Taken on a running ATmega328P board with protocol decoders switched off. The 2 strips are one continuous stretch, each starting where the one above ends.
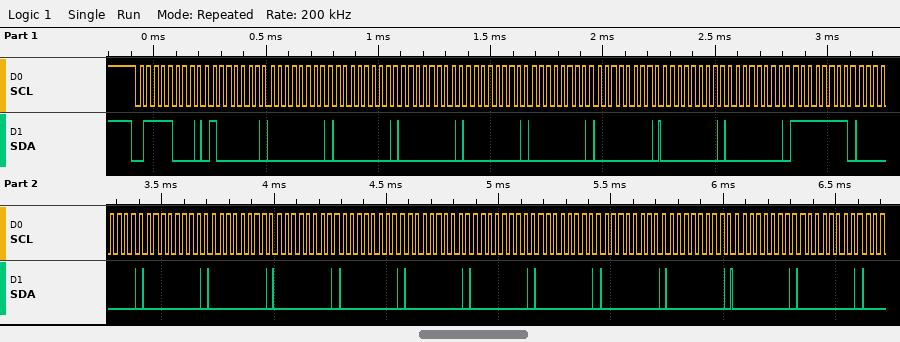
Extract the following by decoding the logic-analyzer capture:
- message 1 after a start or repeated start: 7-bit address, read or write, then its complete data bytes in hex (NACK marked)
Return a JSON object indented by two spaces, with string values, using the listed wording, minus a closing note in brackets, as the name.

{
  "message 1 after a start or repeated start: 7-bit address, read or write, then its complete data bytes in hex": "0x3C write: 40 00 00 00 00 00 00 00 00 FF 00 00 00 00 00 00 00 00 00 00 00 00"
}
